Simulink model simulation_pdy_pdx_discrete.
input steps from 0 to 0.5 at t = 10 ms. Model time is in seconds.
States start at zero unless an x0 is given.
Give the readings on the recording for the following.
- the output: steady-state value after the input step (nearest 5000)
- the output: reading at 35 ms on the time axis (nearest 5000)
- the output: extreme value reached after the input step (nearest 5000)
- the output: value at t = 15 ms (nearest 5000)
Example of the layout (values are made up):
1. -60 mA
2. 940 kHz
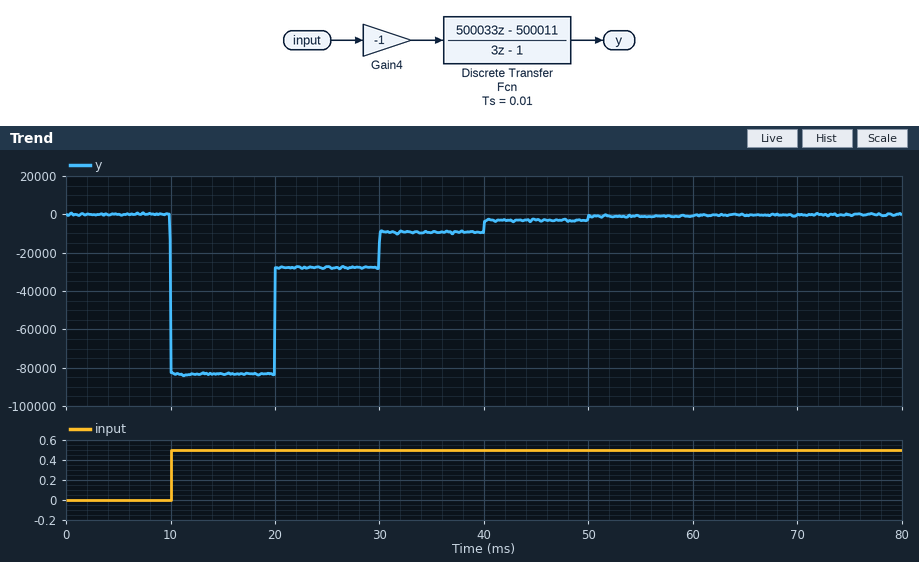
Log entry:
1. 0
2. -10000
3. -85000
4. -85000
